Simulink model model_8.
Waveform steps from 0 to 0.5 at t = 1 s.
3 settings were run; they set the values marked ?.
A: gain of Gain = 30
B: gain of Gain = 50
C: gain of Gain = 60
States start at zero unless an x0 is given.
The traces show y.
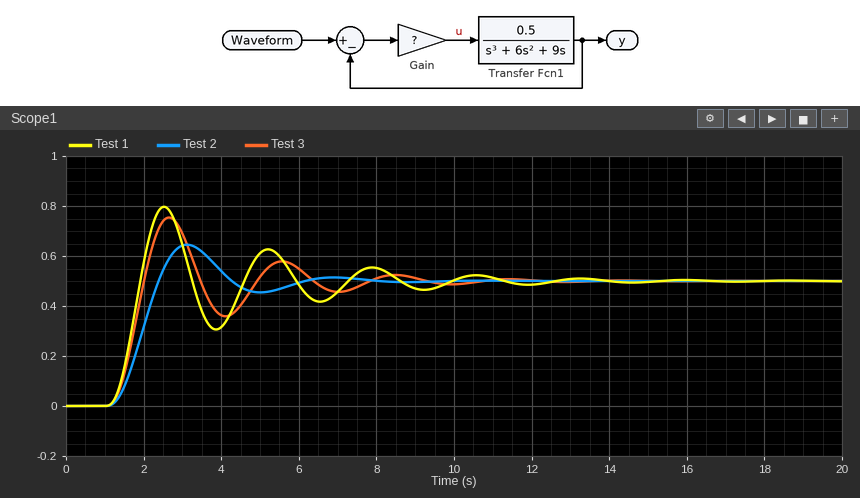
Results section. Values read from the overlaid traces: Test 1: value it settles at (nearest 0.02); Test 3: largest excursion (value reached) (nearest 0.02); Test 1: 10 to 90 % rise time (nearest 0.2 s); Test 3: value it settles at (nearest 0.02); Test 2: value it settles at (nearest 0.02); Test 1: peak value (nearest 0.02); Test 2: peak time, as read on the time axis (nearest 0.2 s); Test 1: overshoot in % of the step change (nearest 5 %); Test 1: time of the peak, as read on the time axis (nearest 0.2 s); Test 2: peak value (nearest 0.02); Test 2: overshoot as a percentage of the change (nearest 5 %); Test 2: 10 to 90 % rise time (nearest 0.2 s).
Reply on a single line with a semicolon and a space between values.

0.50; 0.76; 0.6 s; 0.50; 0.50; 0.80; 3.2 s; 60 %; 2.6 s; 0.64; 30 %; 0.8 s
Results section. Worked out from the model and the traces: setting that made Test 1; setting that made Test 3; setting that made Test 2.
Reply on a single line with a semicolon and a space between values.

C; B; A
